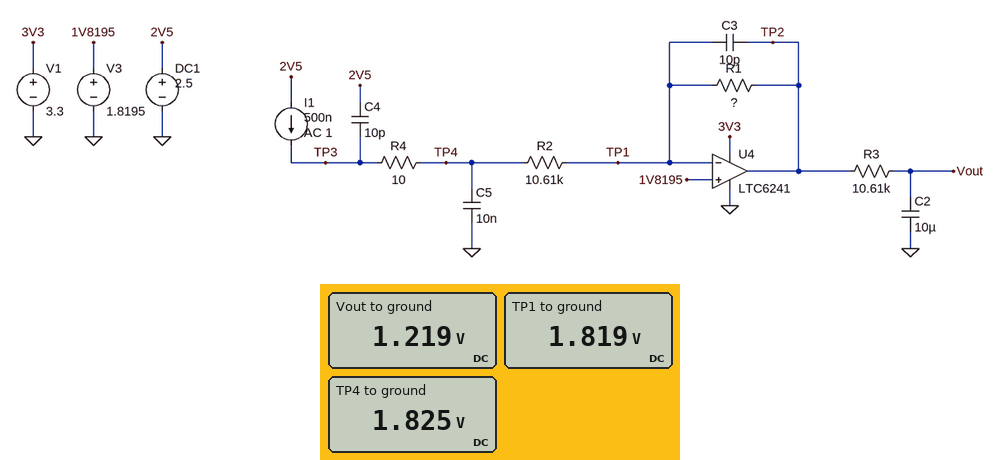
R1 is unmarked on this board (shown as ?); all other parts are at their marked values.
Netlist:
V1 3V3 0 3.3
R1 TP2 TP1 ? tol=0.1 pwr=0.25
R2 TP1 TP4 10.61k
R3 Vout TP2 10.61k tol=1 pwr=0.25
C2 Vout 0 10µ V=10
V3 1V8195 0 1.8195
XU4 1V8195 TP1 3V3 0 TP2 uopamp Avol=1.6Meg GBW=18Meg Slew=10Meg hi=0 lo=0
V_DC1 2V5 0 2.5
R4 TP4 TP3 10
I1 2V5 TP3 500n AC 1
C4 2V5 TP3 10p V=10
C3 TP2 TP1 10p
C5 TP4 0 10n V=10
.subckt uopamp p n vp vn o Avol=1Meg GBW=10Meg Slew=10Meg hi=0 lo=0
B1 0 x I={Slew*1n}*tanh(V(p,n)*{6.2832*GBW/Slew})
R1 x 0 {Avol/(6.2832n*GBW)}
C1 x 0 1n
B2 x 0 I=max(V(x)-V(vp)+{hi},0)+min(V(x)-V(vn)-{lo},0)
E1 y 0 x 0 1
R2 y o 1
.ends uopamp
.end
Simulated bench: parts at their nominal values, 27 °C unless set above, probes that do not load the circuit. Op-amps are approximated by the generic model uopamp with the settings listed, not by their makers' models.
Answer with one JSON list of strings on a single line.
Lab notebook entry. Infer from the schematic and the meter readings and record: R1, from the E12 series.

["1.2 MΩ"]
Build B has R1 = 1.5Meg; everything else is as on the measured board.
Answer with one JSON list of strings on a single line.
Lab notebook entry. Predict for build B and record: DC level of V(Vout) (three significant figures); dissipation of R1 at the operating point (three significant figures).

["1.07 V", "375 nW"]
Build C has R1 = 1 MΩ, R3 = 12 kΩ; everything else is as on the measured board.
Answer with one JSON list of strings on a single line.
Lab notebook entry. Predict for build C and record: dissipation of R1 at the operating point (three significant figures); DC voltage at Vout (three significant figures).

["250 nW", "1.32 V"]
